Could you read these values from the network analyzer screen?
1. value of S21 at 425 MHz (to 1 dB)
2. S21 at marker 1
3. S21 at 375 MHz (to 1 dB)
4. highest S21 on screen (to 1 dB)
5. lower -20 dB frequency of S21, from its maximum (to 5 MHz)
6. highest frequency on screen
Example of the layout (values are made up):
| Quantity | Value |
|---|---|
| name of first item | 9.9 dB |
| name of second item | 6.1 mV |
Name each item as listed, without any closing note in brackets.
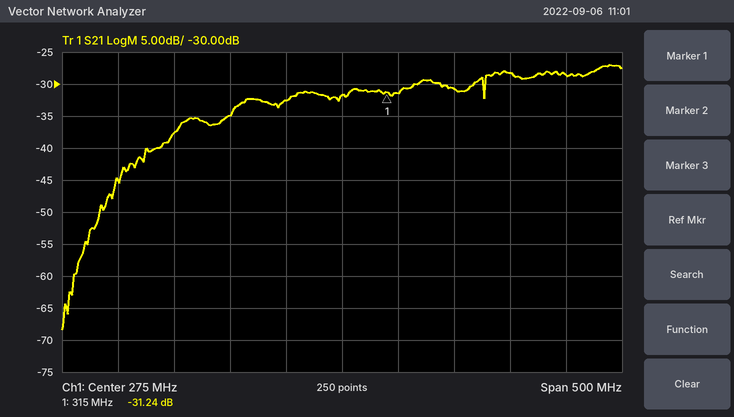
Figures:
| Quantity | Value |
|---|---|
| value of S21 at 425 MHz | -28 dB |
| S21 at marker 1 | -31.24 dB |
| S21 at 375 MHz | -31 dB |
| highest S21 on screen | -27 dB |
| lower -20 dB frequency of S21, from its maximum | 70 MHz |
| highest frequency on screen | 525 MHz |
